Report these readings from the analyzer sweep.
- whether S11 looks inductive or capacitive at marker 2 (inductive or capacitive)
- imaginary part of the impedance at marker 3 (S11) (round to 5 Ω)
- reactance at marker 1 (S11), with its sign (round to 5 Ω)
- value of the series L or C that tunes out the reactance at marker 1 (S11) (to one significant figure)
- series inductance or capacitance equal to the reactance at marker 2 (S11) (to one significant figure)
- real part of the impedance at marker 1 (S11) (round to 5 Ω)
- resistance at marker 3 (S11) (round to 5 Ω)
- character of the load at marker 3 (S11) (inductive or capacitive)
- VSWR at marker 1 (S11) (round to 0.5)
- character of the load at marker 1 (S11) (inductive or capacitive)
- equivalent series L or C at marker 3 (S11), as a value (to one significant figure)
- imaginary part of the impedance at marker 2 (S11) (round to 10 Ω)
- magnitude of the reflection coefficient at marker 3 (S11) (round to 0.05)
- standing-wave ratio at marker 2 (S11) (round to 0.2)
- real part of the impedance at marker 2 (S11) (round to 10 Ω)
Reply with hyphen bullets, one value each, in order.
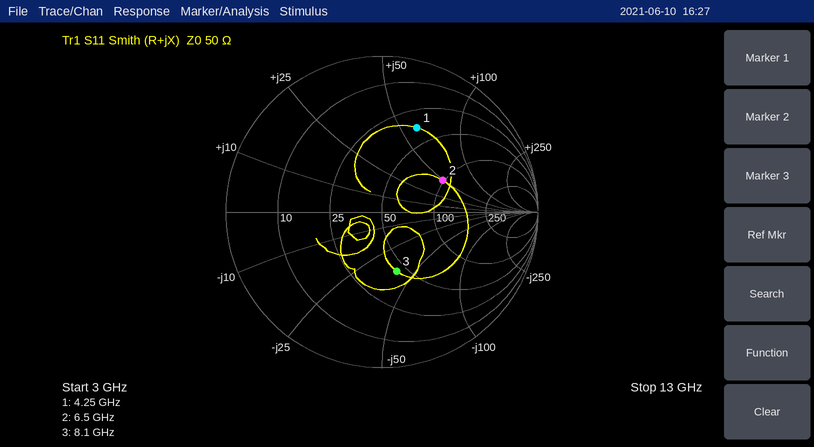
- inductive
- -40 Ω
- +60 Ω
- 600 fF
- 1 nH
- 35 Ω
- 45 Ω
- capacitive
- 4.0
- inductive
- 500 fF
- +50 Ω
- 0.40
- 2.6
- 100 Ω
